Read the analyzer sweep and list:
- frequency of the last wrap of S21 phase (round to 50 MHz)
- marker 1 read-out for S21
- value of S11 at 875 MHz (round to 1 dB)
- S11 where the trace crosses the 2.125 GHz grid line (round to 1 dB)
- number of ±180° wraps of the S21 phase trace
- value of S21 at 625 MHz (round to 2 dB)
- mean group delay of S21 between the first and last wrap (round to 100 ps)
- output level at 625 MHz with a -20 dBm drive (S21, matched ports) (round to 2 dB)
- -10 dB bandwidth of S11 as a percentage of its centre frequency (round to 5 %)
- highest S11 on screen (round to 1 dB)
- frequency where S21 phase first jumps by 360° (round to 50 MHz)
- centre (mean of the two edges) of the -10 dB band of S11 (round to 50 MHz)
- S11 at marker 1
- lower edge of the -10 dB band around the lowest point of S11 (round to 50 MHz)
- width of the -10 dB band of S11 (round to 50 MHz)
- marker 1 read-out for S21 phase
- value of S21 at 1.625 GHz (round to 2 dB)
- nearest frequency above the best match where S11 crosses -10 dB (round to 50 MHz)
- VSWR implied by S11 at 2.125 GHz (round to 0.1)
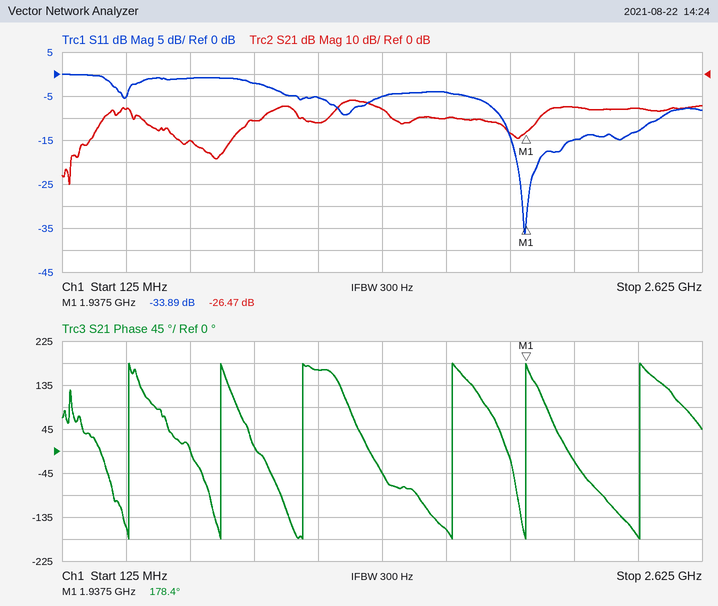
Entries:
2.40 GHz
-26.47 dB
-2 dB
-15 dB
6
-30 dB
2.5 ns
-50 dBm
30 %
0 dB
400 MHz
2.15 GHz
-33.89 dB
1.85 GHz
600 MHz
178.4°
-20 dB
2.45 GHz
1.4
